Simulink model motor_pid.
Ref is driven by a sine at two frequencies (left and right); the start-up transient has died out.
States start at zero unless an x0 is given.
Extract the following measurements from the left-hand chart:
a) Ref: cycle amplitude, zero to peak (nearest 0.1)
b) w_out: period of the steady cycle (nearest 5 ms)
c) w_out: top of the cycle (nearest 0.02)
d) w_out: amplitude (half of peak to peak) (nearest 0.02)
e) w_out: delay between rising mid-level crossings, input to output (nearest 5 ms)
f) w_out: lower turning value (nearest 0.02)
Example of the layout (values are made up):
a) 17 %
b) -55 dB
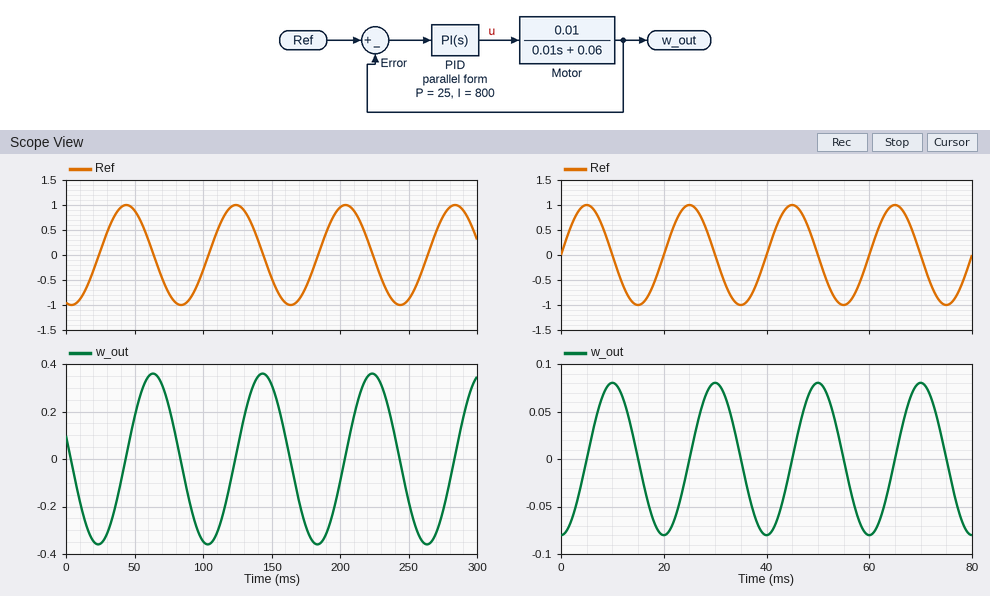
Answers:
a) 1.0
b) 80 ms
c) 0.36
d) 0.36
e) 20 ms
f) -0.36
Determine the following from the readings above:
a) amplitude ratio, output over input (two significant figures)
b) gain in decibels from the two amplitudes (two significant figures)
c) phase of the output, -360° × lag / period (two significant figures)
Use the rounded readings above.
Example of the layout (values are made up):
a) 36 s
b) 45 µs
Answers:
a) 0.36
b) -8.9 dB
c) -90°
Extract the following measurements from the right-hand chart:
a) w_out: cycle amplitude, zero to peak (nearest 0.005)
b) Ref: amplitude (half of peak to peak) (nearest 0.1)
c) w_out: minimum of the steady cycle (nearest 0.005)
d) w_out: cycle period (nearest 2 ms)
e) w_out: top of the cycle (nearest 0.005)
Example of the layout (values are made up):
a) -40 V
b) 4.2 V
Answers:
a) 0.080
b) 1.0
c) -0.080
d) 20 ms
e) 0.080
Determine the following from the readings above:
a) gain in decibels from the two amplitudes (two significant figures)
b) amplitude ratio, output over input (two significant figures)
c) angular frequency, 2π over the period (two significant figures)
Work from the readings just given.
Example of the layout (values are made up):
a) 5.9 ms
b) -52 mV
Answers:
a) -22 dB
b) 0.080
c) 0.31 rad/ms
